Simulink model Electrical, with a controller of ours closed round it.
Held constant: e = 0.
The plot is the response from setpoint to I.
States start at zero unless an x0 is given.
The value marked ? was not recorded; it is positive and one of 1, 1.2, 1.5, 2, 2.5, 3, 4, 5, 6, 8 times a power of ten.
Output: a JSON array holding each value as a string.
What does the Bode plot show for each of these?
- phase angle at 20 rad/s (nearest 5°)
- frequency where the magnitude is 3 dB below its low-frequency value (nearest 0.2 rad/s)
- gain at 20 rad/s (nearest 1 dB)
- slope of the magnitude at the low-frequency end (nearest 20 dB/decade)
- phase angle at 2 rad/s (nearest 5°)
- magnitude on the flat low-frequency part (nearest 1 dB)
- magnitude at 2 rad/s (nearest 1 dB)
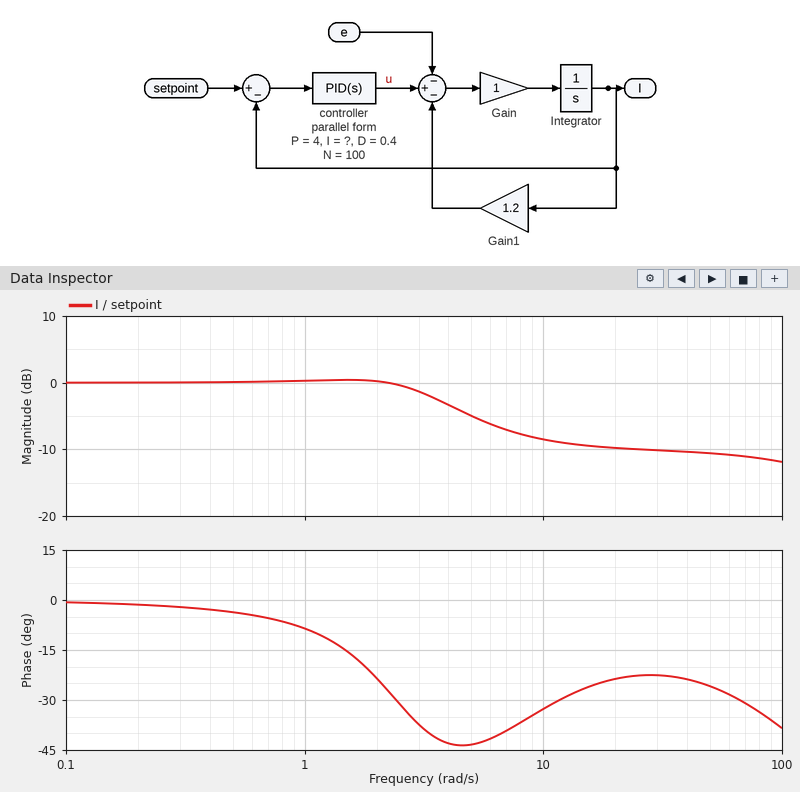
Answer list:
["-25°", "3.8 rad/s", "-10 dB", "0 dB/decade", "-25°", "0 dB", "0 dB"]
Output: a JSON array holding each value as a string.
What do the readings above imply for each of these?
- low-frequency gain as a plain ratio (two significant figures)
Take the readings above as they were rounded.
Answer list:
["1.0"]
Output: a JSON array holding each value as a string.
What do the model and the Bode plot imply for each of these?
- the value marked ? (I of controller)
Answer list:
["10"]
